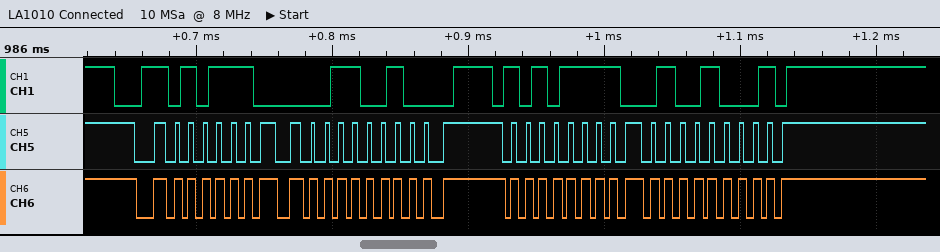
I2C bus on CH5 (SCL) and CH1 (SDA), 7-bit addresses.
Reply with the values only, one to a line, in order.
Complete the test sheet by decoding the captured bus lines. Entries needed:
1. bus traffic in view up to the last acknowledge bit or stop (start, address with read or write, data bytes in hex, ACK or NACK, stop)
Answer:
start, address 57 write ACK, 32 ACK, stop, start, address 57 read ACK, 48 NACK, stop
